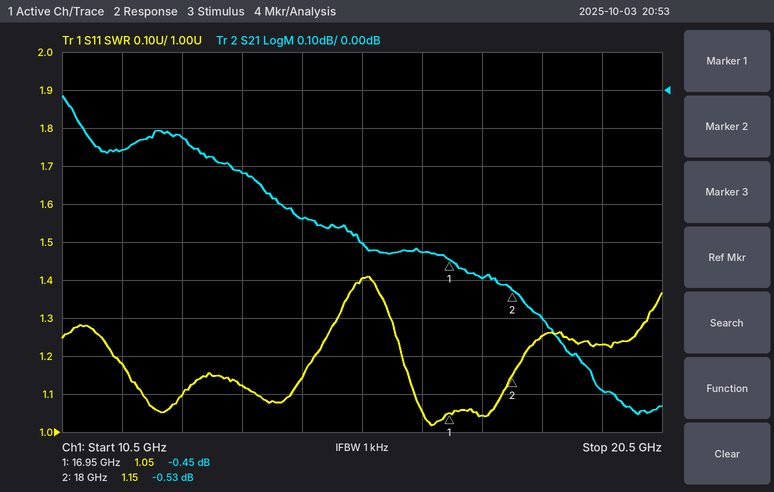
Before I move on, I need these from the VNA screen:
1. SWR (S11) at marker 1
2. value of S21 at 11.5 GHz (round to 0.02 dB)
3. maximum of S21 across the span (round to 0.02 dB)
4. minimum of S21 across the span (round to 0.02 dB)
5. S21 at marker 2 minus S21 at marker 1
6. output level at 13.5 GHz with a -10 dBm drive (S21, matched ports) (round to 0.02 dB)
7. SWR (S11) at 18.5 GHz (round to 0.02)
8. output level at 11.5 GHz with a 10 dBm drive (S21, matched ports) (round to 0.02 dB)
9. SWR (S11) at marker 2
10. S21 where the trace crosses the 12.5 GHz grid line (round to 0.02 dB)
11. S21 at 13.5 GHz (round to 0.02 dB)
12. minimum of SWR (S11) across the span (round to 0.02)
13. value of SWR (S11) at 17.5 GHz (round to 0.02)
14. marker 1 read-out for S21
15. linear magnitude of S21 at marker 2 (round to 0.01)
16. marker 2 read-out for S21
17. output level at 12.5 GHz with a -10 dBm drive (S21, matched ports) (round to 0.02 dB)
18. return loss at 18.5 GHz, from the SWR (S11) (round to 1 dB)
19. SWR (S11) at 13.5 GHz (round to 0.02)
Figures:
1.05
-0.16 dB
-0.02 dB
-0.86 dB
-0.08 dB
-10.22 dBm
1.26
9.84 dBm
1.15
-0.12 dB
-0.22 dB
1.02
1.04
-0.45 dB
0.94
-0.53 dB
-10.12 dBm
19 dB
1.12
